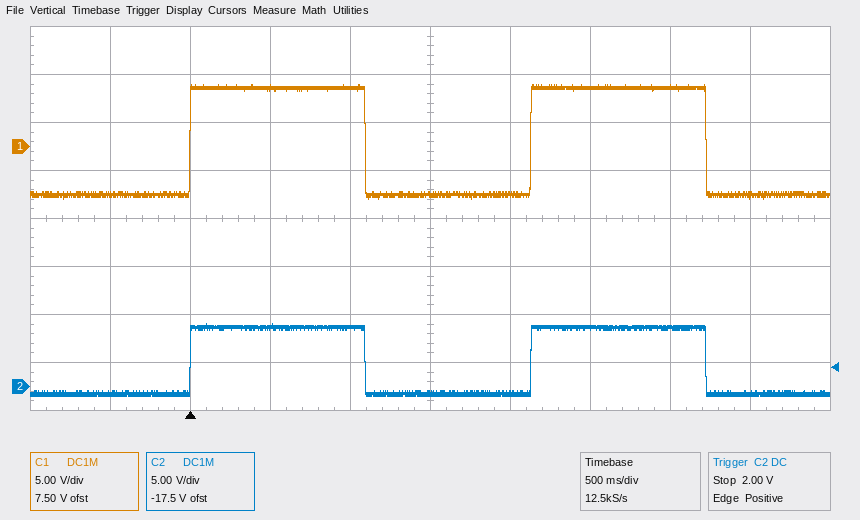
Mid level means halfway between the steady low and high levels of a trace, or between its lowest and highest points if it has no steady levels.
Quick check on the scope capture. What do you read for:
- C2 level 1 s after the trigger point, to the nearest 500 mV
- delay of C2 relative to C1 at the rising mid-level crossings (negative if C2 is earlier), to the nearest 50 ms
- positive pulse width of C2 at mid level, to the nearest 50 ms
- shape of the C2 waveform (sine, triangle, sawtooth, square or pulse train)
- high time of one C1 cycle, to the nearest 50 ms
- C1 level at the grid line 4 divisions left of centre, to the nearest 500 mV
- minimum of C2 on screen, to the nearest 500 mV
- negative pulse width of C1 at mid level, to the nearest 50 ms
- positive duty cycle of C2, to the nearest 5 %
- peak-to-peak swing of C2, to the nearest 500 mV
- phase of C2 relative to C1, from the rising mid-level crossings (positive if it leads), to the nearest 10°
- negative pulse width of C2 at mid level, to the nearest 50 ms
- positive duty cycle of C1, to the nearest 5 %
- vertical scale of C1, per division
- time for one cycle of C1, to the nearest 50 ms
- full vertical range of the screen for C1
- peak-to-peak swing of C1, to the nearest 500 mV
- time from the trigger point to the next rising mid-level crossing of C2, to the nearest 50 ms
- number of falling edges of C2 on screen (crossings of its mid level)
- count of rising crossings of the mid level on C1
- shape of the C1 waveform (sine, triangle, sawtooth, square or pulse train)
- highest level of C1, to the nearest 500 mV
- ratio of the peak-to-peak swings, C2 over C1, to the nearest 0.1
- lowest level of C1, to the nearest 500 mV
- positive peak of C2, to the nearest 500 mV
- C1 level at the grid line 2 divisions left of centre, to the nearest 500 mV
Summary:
6.0 V
0 ms
1.10 s
square
1.10 s
-5.0 V
-1.0 V
1.05 s
50 %
7.5 V
0°
1.05 s
50 %
5 V
2.15 s
40 V
12.0 V
2.15 s
2
2
square
6.5 V
0.6
-5.5 V
6.5 V
6.0 V
